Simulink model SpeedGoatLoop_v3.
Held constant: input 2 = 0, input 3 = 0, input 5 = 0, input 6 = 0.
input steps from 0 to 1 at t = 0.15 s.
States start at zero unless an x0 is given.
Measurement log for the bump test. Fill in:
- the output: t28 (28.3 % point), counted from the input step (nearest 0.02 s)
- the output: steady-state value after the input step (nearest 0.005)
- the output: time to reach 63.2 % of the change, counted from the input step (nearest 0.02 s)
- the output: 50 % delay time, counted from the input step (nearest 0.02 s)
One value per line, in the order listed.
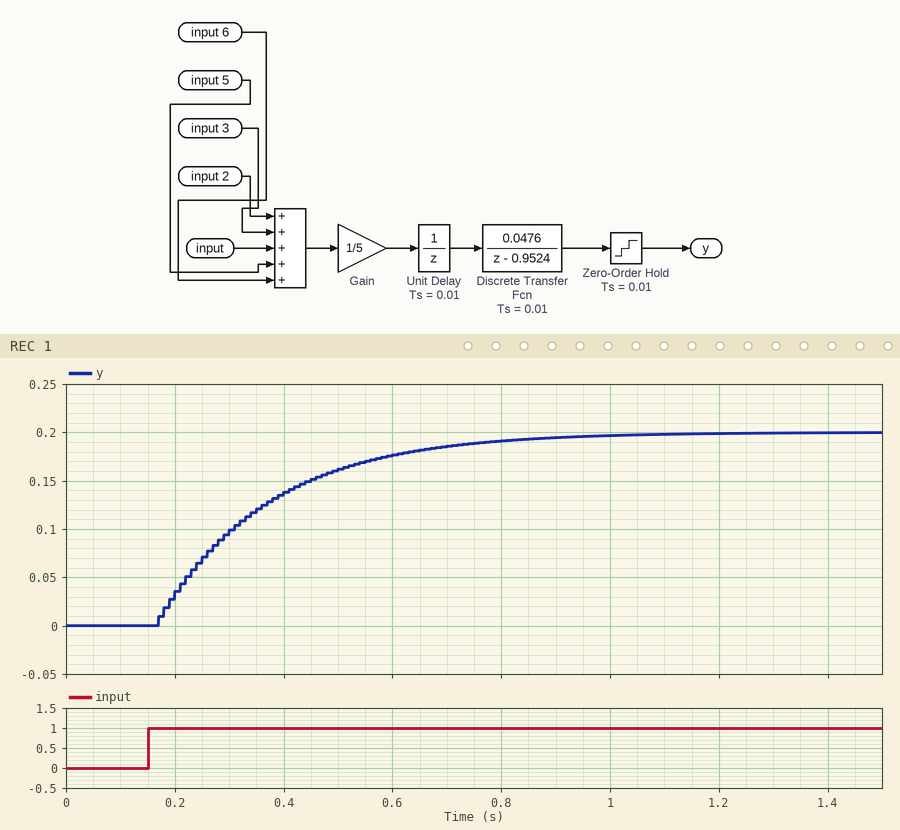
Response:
0.08 s
0.200
0.22 s
0.16 s
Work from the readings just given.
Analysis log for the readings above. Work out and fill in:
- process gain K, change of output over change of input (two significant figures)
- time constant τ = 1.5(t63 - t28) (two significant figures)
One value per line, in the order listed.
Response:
0.20
0.21 s
